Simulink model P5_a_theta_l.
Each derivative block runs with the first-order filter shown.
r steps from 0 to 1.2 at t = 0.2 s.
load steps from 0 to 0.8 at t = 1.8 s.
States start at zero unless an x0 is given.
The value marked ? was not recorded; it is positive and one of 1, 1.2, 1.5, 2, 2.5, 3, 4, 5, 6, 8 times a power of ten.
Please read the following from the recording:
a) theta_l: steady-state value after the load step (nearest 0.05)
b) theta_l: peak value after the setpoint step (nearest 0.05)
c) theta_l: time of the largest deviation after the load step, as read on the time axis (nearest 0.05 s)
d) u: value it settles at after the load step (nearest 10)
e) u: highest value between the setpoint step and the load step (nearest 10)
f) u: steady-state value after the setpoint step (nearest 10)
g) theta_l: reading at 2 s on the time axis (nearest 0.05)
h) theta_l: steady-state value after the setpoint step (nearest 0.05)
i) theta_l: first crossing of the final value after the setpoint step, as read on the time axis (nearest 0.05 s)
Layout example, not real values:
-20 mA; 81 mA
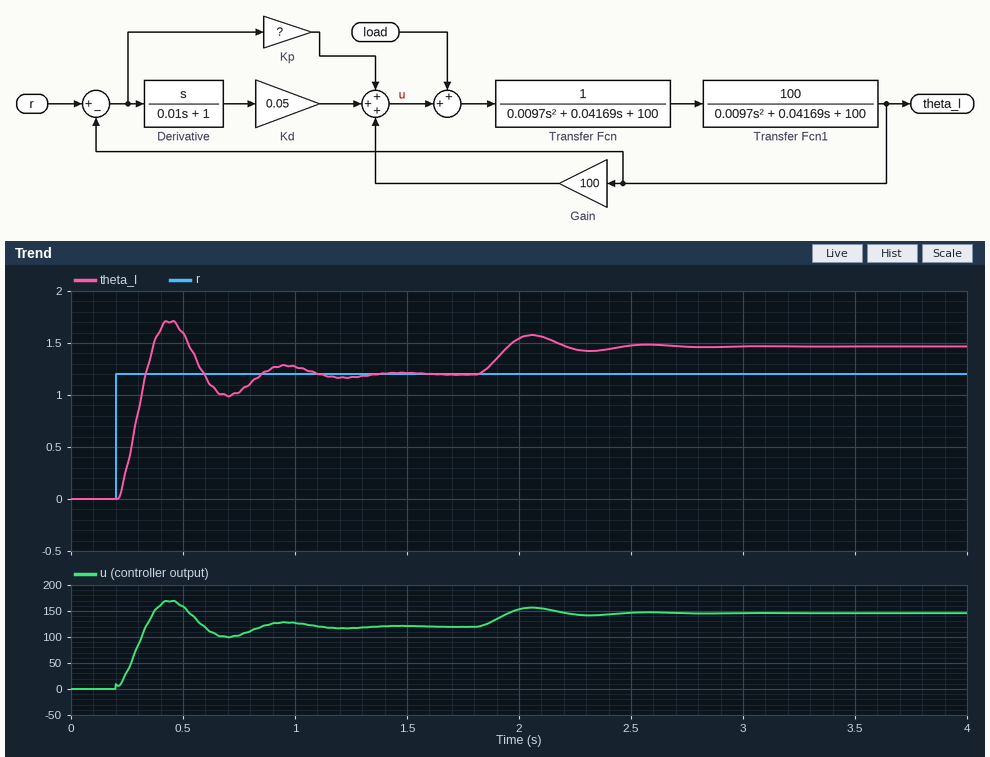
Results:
1.45; 1.70; 2.05 s; 150; 170; 120; 1.55; 1.20; 0.35 s
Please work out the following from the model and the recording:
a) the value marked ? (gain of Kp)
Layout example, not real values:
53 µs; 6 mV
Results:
3
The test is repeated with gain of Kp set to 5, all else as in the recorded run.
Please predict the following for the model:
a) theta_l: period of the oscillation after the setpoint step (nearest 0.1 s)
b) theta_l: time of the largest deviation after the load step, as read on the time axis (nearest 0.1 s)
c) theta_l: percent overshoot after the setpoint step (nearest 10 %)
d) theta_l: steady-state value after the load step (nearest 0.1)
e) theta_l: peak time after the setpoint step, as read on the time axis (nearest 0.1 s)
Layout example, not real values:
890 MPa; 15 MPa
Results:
0.4 s; 2.0 s; 50 %; 1.4; 0.4 s
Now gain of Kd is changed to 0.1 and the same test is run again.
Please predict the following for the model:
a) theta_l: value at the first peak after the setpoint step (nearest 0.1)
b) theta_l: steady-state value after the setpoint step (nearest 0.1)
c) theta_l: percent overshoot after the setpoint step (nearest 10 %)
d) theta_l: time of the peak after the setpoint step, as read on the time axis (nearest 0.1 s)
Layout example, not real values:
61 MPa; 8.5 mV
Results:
1.6; 1.2; 30 %; 0.4 s
